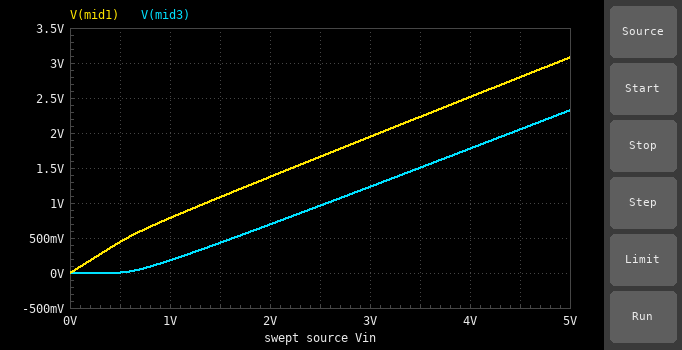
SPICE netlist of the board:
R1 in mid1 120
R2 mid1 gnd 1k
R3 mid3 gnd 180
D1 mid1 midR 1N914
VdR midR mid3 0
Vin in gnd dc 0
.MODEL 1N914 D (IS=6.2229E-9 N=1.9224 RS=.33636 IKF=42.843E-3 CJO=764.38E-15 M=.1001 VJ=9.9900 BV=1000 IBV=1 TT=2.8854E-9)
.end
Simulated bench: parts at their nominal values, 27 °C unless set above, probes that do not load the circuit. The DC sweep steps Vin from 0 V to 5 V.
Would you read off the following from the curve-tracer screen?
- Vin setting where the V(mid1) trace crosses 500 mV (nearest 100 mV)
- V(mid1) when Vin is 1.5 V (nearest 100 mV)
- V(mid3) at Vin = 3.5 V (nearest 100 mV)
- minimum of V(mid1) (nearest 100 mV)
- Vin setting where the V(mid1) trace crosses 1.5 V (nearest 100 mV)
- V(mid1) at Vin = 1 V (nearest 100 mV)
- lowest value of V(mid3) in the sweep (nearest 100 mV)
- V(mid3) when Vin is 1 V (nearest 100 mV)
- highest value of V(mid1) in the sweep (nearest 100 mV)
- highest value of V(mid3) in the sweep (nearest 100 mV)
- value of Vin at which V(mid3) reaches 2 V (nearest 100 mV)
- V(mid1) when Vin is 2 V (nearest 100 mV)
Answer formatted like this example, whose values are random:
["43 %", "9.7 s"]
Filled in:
["600 mV", "1.1 V", "1.5 V", "0 V", "2.2 V", "800 mV", "0 V", "200 mV", "3.1 V", "2.3 V", "4.4 V", "1.4 V"]
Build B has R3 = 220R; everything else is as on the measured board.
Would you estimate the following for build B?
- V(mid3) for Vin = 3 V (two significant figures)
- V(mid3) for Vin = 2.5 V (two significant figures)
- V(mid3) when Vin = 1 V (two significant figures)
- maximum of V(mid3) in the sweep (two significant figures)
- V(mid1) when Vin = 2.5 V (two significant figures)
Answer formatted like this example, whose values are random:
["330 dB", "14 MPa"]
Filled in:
["1.3 V", "1.0 V", "200 mV", "2.5 V", "1.7 V"]
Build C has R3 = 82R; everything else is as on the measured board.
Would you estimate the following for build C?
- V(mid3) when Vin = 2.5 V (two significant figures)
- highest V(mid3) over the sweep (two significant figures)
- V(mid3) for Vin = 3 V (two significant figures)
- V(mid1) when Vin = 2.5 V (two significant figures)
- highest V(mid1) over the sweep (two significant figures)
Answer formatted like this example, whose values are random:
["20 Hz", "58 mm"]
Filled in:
["650 mV", "1.6 V", "840 mV", "1.4 V", "2.4 V"]
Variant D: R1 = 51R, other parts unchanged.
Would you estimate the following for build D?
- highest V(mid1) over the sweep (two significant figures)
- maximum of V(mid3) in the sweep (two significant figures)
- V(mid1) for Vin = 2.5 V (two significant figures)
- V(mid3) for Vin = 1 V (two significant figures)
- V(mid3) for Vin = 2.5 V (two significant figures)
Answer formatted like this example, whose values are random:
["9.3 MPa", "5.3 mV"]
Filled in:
["3.9 V", "3.1 V", "2.0 V", "260 mV", "1.3 V"]
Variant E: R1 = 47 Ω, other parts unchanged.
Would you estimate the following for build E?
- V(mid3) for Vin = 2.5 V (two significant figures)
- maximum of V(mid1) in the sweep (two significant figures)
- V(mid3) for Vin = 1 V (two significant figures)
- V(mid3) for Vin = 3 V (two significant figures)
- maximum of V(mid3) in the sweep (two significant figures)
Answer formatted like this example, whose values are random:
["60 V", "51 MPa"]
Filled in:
["1.3 V", "4.0 V", "260 mV", "1.7 V", "3.2 V"]
